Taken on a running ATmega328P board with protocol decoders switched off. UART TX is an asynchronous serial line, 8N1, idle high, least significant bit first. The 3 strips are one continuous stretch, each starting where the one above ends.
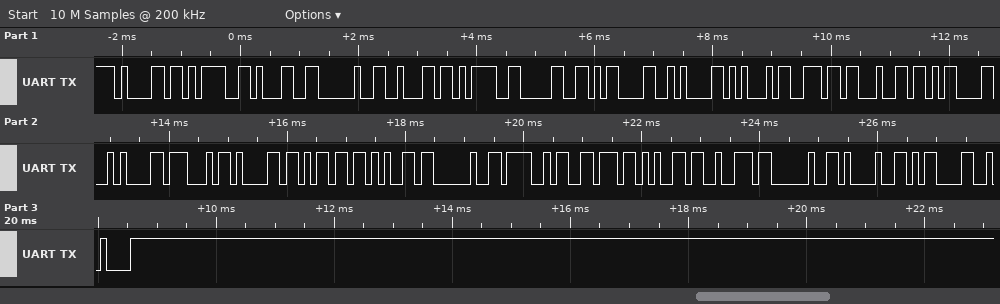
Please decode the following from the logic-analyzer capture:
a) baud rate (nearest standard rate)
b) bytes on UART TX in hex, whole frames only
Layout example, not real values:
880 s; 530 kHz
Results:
9600 baud; 61 3D 31 20 62 3D 30 0D 0A 45 6E 64 0D 0A 47 61 6D 65 20 4F 76 65 72 20 21 0D 0A
